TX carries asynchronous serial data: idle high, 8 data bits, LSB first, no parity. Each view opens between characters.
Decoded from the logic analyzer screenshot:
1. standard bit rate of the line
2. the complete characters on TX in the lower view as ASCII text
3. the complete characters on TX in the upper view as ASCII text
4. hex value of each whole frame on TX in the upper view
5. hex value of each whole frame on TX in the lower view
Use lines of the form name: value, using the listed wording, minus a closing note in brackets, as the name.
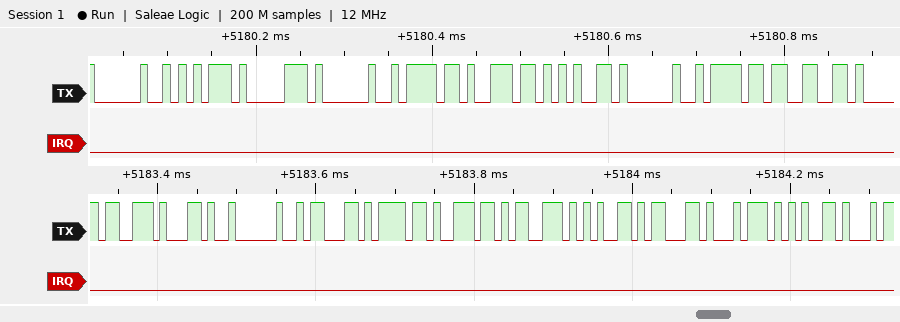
standard bit rate of the line: 115200 baud
the complete characters on TX in the lower view as ASCII text: "s, consecte"
the complete characters on TX in the upper view as ASCII text: " up one of"
hex value of each whole frame on TX in the upper view: 20, 75, 70, 20, 6F, 6E, 65, 20, 6F, 66
hex value of each whole frame on TX in the lower view: 73, 2C, 20, 63, 6F, 6E, 73, 65, 63, 74, 65
